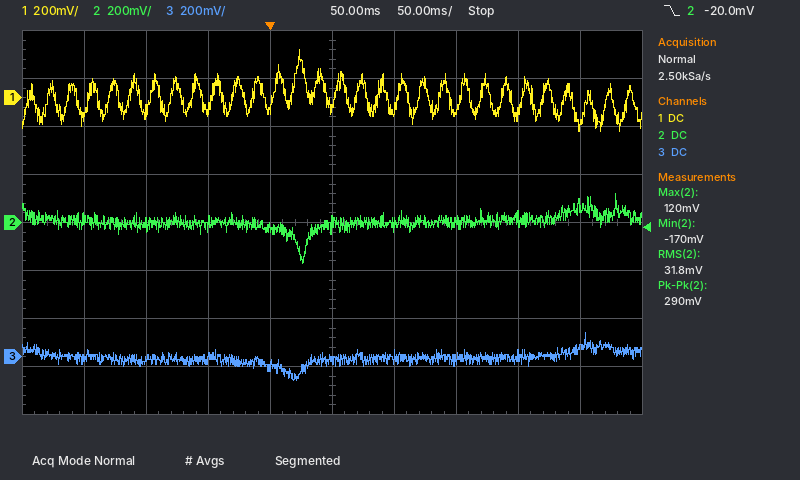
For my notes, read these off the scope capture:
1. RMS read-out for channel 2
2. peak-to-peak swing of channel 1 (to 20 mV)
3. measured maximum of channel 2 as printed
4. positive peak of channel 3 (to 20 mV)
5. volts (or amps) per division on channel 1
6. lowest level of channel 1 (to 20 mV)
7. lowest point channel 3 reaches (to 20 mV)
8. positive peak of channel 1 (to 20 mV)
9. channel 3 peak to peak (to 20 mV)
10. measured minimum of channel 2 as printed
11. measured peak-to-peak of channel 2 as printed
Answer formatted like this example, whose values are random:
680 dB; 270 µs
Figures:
31.8 mV; 340 mV; 120 mV; 100 mV; 200 mV; -140 mV; -100 mV; 200 mV; 200 mV; -170 mV; 290 mV
